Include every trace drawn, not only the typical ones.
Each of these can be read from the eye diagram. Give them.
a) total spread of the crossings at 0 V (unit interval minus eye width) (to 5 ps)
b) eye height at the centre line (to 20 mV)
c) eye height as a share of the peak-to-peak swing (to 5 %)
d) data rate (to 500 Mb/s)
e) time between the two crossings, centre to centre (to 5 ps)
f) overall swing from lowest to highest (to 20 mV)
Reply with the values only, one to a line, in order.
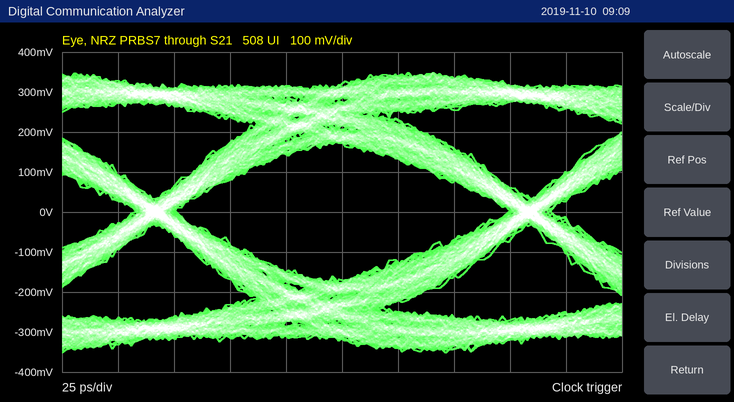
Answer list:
20 ps
340 mV
50 %
6.0 Gb/s
165 ps
700 mV
